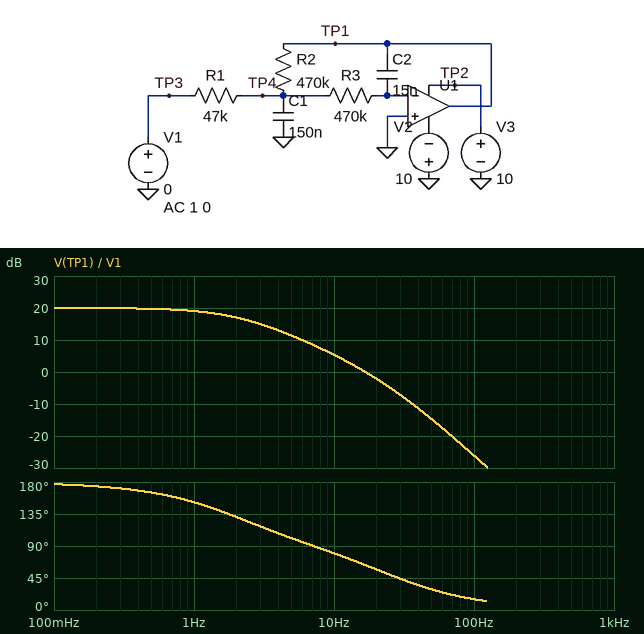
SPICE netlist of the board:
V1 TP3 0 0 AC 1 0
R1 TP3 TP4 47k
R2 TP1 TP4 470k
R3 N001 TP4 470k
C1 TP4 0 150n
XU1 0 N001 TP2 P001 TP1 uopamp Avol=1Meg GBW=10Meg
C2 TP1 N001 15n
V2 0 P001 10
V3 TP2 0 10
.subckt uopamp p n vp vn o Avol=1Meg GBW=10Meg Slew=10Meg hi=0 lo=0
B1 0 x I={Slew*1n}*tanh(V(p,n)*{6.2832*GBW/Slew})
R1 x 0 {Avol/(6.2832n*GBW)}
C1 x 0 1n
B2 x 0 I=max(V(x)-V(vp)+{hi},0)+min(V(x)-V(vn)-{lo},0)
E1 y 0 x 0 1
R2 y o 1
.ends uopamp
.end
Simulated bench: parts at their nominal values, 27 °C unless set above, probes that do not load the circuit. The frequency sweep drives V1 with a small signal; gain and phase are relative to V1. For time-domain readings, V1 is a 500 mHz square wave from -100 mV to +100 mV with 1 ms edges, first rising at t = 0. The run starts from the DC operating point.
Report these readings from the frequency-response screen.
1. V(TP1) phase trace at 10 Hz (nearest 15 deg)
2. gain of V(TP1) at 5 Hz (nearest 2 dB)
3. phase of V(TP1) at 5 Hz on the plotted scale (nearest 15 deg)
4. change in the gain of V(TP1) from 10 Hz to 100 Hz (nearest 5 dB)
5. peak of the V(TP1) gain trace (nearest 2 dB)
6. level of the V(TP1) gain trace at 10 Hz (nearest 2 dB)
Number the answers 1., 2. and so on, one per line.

1. 75 deg
2. 12 dB
3. 105 deg
4. -30 dB
5. 20 dB
6. 6 dB
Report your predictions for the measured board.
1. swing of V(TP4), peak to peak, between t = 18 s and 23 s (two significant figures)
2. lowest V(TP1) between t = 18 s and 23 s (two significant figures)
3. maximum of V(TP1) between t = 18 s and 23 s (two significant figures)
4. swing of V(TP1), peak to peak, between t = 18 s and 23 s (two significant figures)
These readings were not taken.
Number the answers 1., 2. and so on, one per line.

1. 290 mV
2. -1.0 V
3. 1.0 V
4. 2.0 V
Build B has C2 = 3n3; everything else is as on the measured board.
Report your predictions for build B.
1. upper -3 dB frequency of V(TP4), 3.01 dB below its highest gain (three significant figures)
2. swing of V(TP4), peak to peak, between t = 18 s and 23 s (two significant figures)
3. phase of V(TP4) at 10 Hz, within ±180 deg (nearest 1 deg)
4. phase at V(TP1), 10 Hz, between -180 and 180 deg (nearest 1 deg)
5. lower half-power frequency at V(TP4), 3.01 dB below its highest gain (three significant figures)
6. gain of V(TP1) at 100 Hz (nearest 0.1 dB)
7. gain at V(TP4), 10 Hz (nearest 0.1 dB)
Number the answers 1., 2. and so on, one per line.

1. 33.9 Hz
2. 240 mV
3. 26 deg
4. 116 deg
5. 6.83 Hz
6. -12.8 dB
7. -2.5 dB
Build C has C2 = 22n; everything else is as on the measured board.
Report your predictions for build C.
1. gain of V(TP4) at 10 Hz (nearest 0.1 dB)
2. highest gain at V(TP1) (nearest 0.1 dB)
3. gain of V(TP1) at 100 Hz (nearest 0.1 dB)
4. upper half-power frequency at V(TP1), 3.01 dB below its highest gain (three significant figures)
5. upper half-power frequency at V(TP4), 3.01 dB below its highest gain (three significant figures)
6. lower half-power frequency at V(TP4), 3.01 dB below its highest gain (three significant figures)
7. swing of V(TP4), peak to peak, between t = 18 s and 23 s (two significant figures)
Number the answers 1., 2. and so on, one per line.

1. -1.8 dB
2. 20.0 dB
3. -29.5 dB
4. 1.35 Hz
5. 28.3 Hz
6. 1.23 Hz
7. 300 mV
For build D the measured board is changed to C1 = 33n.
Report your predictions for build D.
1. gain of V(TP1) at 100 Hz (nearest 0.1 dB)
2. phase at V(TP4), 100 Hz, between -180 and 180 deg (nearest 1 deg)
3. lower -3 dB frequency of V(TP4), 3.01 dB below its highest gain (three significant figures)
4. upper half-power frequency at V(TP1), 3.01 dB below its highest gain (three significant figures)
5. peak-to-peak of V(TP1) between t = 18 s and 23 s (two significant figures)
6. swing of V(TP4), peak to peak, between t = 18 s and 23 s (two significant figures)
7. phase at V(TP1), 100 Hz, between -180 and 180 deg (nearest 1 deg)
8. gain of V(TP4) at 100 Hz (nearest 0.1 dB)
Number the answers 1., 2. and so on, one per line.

1. -16.6 dB
2. -38 deg
3. 1.85 Hz
4. 1.91 Hz
5. 2.0 V
6. 320 mV
7. 52 deg
8. -3.7 dB
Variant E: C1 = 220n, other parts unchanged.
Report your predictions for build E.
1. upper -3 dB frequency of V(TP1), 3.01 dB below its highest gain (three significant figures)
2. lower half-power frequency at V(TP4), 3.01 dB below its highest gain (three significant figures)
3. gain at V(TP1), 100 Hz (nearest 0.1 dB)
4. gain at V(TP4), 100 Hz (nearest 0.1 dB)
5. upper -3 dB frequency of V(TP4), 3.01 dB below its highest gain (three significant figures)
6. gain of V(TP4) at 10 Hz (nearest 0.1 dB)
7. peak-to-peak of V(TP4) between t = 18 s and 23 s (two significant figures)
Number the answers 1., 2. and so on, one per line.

1. 2.09 Hz
2. 1.72 Hz
3. -29.3 dB
4. -16.4 dB
5. 20.2 Hz
6. -2.1 dB
7. 280 mV
